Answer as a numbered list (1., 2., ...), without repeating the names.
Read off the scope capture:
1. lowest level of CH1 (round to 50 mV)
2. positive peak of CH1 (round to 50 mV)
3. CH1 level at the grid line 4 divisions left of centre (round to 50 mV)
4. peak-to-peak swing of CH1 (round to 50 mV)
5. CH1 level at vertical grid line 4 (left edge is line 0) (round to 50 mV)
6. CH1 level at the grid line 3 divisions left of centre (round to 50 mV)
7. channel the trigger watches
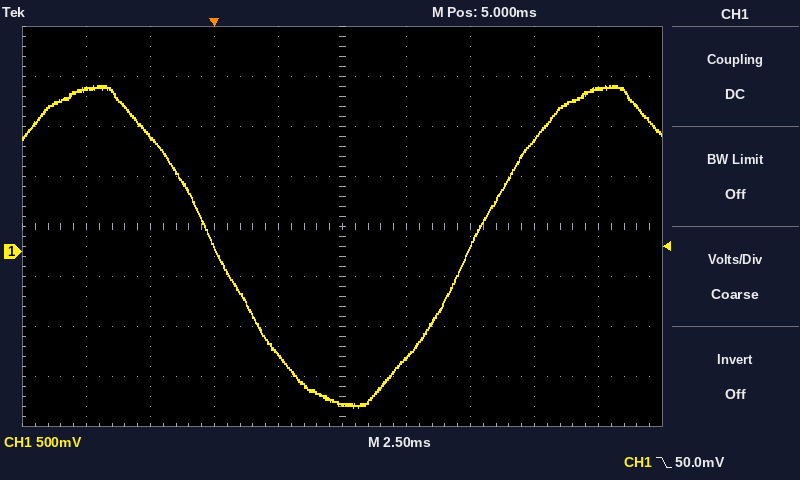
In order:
1. -1.55 V
2. 1.65 V
3. 1.60 V
4. 3.20 V
5. -1.00 V
6. 1.15 V
7. CH1
